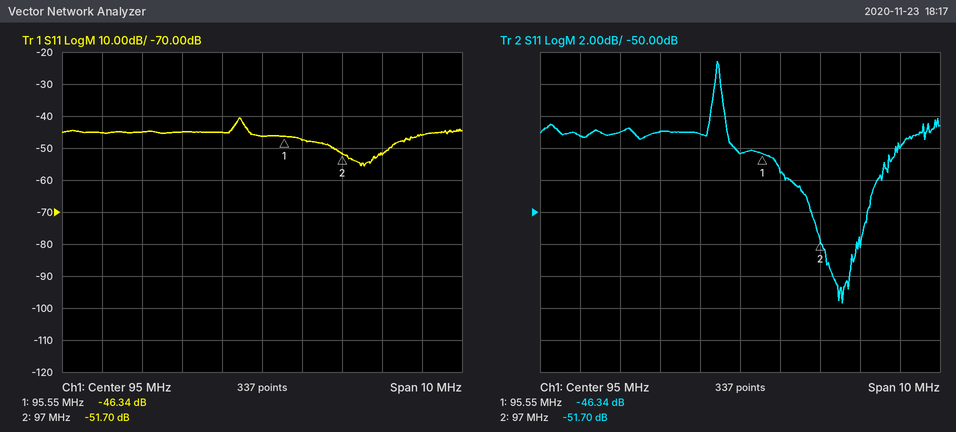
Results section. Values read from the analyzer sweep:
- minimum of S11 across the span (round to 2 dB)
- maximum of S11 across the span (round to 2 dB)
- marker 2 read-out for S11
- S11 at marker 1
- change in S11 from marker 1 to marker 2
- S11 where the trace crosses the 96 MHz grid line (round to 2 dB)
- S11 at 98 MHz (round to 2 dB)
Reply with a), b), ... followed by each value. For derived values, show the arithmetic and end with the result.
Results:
a) -56 dB
b) -40 dB
c) -51.70 dB
d) -46.34 dB
e) -51.7 − (-46.34) = -5.36 dB
f) -48 dB
g) -52 dB
